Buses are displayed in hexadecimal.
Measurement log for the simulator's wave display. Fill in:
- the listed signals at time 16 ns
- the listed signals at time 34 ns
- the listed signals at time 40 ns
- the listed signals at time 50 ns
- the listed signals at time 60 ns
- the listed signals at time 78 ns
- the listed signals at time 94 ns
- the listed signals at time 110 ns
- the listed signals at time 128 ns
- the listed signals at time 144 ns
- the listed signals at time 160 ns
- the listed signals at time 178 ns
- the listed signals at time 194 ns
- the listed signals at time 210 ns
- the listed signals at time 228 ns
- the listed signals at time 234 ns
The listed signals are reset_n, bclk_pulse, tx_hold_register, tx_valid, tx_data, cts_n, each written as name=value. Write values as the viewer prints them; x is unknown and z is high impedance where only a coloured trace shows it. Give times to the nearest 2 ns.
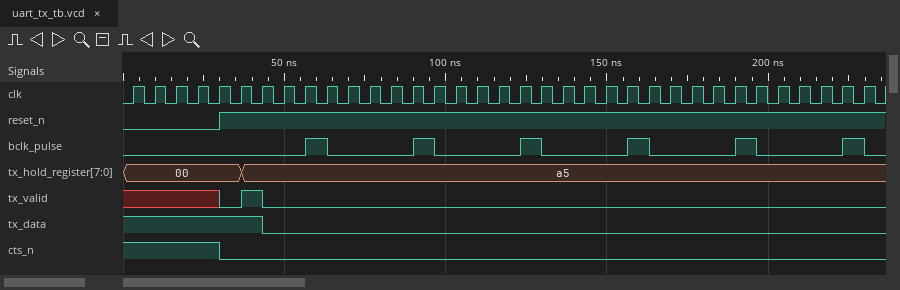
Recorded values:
reset_n=0, bclk_pulse=0, tx_hold_register=00, tx_valid=x, tx_data=1, cts_n=1
reset_n=1, bclk_pulse=0, tx_hold_register=00, tx_valid=0, tx_data=1, cts_n=0
reset_n=1, bclk_pulse=0, tx_hold_register=a5, tx_valid=1, tx_data=1, cts_n=0
reset_n=1, bclk_pulse=0, tx_hold_register=a5, tx_valid=0, tx_data=0, cts_n=0
reset_n=1, bclk_pulse=1, tx_hold_register=a5, tx_valid=0, tx_data=0, cts_n=0
reset_n=1, bclk_pulse=0, tx_hold_register=a5, tx_valid=0, tx_data=0, cts_n=0
reset_n=1, bclk_pulse=1, tx_hold_register=a5, tx_valid=0, tx_data=0, cts_n=0
reset_n=1, bclk_pulse=0, tx_hold_register=a5, tx_valid=0, tx_data=0, cts_n=0
reset_n=1, bclk_pulse=1, tx_hold_register=a5, tx_valid=0, tx_data=0, cts_n=0
reset_n=1, bclk_pulse=0, tx_hold_register=a5, tx_valid=0, tx_data=0, cts_n=0
reset_n=1, bclk_pulse=1, tx_hold_register=a5, tx_valid=0, tx_data=0, cts_n=0
reset_n=1, bclk_pulse=0, tx_hold_register=a5, tx_valid=0, tx_data=0, cts_n=0
reset_n=1, bclk_pulse=1, tx_hold_register=a5, tx_valid=0, tx_data=0, cts_n=0
reset_n=1, bclk_pulse=0, tx_hold_register=a5, tx_valid=0, tx_data=0, cts_n=0
reset_n=1, bclk_pulse=1, tx_hold_register=a5, tx_valid=0, tx_data=0, cts_n=0
reset_n=1, bclk_pulse=0, tx_hold_register=a5, tx_valid=0, tx_data=0, cts_n=0
